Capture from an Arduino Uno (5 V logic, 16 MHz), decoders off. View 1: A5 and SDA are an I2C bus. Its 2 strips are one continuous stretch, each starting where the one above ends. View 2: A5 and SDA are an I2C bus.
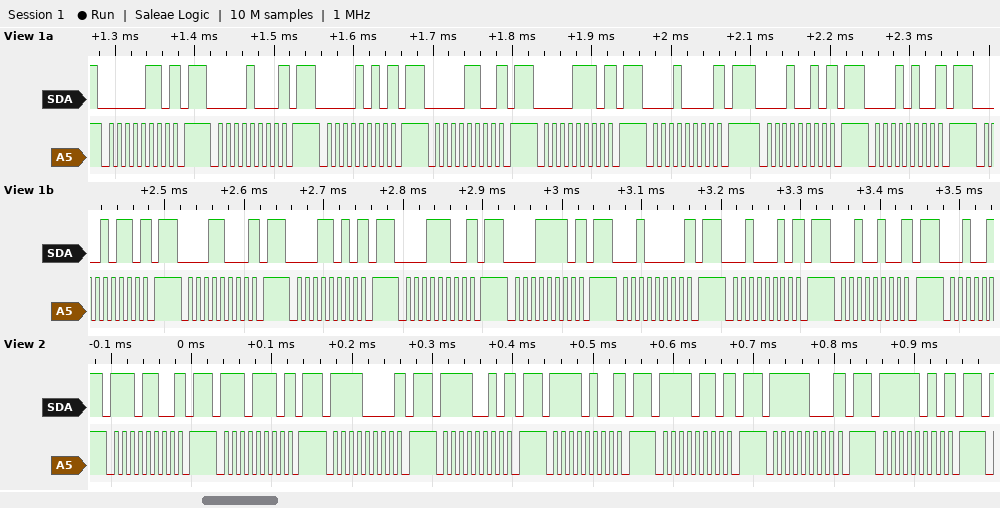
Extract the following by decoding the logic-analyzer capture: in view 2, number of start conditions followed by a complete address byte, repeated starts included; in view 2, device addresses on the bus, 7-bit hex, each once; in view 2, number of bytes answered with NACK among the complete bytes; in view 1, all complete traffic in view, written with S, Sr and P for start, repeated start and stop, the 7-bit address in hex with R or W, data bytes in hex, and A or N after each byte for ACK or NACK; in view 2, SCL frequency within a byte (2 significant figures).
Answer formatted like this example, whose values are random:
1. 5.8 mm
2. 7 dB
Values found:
1. 8
2. 0x76 0x77 0x78 0x79 0x7A 0x7B 0x7C 0x7D
3. 8
4. S 03W N P S 04W N P S 05W N P S 06W N P S 07W N P S 08W N P S 09W N P S 0AW N P S 0BW N P S 0CW N P S 0DW N P S 0EW N P S 0FW N P S 10W N P S 11W N P S 12W N P
5. 100 kHz
